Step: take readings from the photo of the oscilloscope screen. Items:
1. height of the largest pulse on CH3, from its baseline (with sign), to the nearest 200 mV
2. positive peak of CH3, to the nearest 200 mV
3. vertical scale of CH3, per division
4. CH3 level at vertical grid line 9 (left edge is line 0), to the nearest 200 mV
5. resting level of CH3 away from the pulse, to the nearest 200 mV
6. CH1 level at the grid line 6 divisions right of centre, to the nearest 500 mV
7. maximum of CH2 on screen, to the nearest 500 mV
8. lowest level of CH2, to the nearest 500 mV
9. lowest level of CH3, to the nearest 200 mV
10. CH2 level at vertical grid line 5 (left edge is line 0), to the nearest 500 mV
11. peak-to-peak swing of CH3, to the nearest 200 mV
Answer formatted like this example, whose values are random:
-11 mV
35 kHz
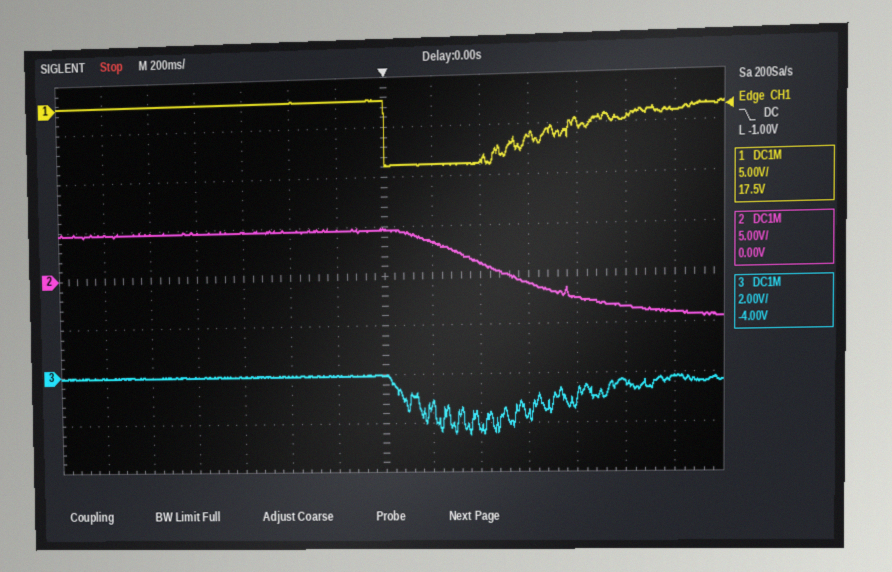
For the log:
-2.4 V
0.0 V
2 V
-2.2 V
0.0 V
-1.5 V
5.0 V
-4.5 V
-2.4 V
4.5 V
2.4 V
